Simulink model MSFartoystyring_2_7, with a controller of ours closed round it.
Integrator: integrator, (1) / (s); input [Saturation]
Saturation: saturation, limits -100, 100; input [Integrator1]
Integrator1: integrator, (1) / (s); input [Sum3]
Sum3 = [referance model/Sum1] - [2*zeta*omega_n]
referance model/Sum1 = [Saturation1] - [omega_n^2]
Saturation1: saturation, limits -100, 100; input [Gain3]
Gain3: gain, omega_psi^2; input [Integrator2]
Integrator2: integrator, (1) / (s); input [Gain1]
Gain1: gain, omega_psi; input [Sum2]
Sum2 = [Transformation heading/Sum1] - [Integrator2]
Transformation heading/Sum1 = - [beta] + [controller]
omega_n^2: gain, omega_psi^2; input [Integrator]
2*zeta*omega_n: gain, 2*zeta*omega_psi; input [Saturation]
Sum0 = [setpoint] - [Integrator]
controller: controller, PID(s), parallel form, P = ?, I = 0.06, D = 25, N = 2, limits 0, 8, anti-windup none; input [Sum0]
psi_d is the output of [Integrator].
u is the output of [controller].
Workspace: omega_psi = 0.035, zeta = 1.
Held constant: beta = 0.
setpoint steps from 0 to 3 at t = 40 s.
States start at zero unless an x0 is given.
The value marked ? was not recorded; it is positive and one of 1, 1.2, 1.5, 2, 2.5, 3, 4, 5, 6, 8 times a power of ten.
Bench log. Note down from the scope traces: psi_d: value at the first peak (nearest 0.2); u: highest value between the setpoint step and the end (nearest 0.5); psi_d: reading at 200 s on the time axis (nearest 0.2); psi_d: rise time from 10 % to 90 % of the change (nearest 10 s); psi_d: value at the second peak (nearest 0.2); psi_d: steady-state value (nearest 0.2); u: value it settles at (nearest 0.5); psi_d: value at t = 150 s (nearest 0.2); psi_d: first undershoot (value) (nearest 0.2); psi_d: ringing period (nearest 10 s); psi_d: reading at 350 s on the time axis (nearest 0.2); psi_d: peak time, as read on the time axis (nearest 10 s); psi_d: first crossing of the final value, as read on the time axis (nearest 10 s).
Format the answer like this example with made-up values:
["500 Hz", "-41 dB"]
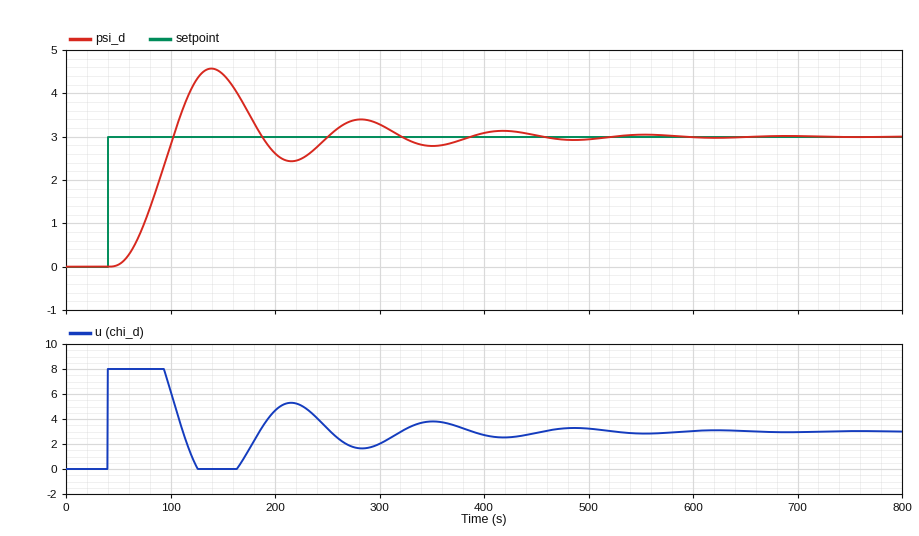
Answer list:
["4.6", "8.0", "2.6", "40 s", "3.4", "3.0", "3.0", "4.4", "2.4", "140 s", "2.8", "140 s", "100 s"]
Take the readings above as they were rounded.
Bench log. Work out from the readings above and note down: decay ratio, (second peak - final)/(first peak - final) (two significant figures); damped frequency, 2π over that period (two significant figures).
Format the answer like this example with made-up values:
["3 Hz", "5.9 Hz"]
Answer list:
["0.25", "0.045 rad/s"]
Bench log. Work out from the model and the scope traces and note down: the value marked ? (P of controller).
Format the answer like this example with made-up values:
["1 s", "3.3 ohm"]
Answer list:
["4"]
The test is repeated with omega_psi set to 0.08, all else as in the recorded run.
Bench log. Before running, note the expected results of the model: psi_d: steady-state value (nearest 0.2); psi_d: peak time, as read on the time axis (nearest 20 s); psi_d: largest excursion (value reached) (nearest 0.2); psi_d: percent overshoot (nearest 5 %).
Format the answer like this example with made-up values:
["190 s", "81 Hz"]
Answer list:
["3.0", "80 s", "3.4", "15 %"]
